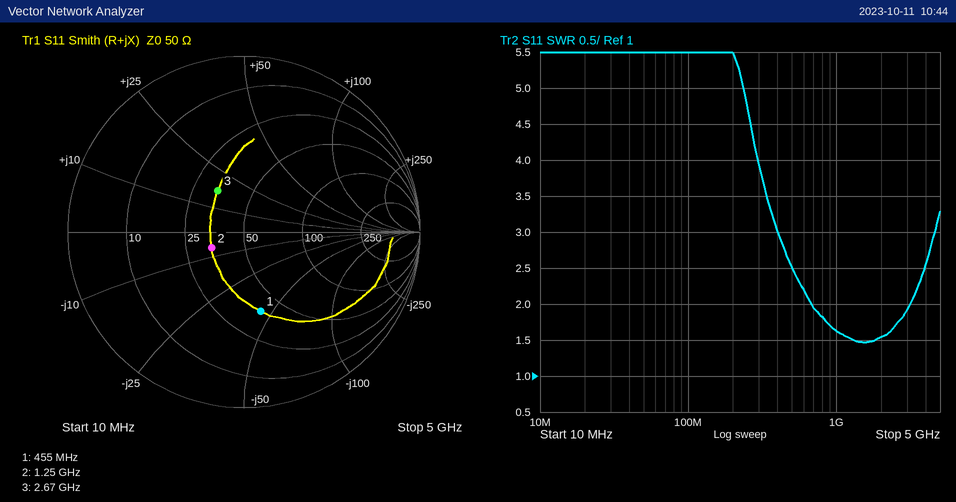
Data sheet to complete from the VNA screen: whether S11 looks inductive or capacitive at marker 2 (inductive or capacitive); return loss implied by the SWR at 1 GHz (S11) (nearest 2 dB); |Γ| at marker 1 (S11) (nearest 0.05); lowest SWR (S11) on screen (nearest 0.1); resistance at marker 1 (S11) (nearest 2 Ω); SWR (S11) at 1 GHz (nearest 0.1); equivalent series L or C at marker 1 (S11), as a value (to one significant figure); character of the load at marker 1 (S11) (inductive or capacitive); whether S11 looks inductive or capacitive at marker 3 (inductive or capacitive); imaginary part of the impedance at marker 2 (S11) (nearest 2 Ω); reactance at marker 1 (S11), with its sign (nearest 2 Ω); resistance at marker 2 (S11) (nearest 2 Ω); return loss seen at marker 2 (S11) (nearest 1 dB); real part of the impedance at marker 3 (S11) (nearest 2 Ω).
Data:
capacitive
12 dB
0.45
1.5
38 Ω
1.6
8 pF
capacitive
inductive
-6 Ω
-44 Ω
34 Ω
14 dB
34 Ω
